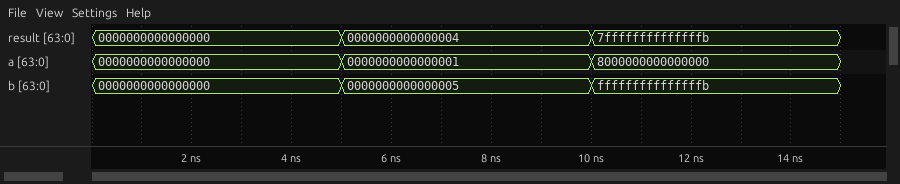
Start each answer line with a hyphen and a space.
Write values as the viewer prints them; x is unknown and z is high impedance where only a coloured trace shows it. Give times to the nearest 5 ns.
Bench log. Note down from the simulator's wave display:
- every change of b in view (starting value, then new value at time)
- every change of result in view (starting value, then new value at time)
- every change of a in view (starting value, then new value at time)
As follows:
- 0000000000000000, 0000000000000005 at 5 ns, fffffffffffffffb at 10 ns
- 0000000000000000, 0000000000000004 at 5 ns, 7ffffffffffffffb at 10 ns
- 0000000000000000, 0000000000000001 at 5 ns, 8000000000000000 at 10 ns
